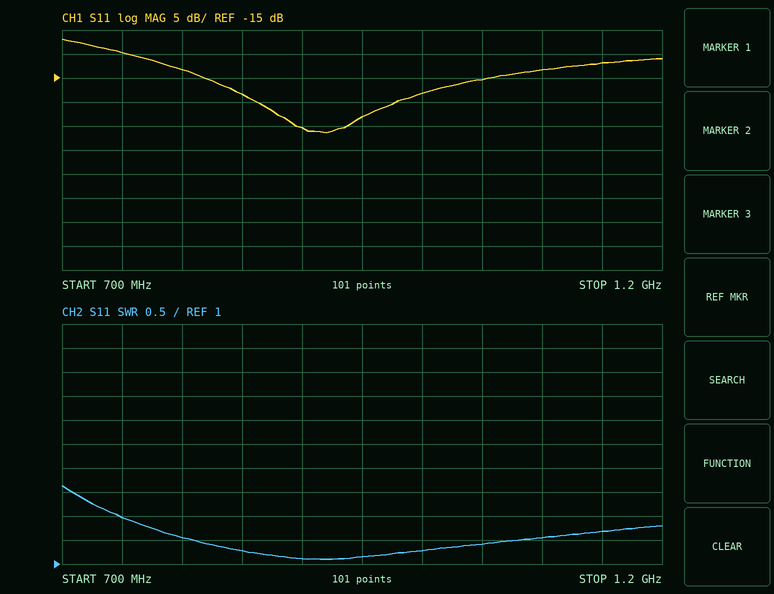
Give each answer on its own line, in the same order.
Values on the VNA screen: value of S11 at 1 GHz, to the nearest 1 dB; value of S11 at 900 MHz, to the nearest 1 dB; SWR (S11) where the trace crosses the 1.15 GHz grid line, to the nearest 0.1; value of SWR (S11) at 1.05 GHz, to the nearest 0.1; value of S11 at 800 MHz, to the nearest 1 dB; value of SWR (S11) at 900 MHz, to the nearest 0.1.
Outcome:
-18 dB
-25 dB
1.7
1.4
-13 dB
1.1
